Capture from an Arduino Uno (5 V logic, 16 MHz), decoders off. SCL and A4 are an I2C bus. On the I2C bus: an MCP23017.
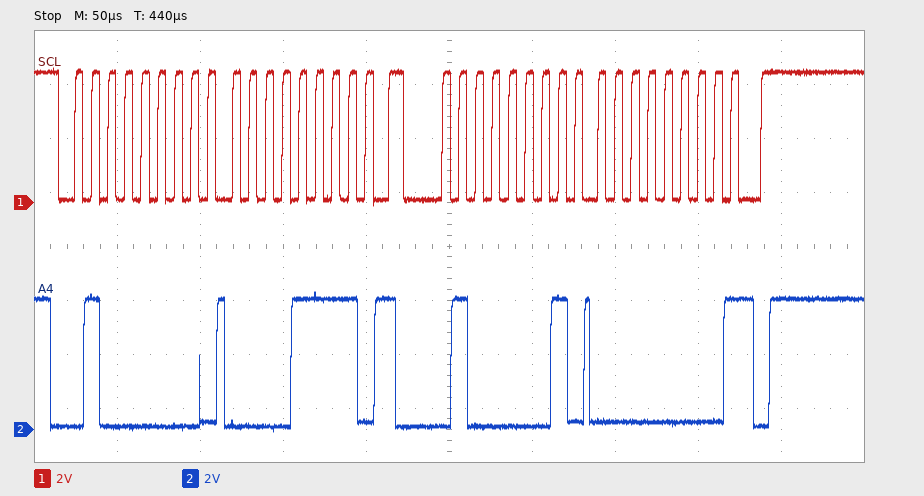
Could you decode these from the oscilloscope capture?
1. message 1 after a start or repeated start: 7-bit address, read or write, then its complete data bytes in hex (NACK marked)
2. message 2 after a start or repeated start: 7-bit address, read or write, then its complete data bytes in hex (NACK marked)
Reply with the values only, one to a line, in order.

0x20 write: 0F
0x20 read: 00 NACK
